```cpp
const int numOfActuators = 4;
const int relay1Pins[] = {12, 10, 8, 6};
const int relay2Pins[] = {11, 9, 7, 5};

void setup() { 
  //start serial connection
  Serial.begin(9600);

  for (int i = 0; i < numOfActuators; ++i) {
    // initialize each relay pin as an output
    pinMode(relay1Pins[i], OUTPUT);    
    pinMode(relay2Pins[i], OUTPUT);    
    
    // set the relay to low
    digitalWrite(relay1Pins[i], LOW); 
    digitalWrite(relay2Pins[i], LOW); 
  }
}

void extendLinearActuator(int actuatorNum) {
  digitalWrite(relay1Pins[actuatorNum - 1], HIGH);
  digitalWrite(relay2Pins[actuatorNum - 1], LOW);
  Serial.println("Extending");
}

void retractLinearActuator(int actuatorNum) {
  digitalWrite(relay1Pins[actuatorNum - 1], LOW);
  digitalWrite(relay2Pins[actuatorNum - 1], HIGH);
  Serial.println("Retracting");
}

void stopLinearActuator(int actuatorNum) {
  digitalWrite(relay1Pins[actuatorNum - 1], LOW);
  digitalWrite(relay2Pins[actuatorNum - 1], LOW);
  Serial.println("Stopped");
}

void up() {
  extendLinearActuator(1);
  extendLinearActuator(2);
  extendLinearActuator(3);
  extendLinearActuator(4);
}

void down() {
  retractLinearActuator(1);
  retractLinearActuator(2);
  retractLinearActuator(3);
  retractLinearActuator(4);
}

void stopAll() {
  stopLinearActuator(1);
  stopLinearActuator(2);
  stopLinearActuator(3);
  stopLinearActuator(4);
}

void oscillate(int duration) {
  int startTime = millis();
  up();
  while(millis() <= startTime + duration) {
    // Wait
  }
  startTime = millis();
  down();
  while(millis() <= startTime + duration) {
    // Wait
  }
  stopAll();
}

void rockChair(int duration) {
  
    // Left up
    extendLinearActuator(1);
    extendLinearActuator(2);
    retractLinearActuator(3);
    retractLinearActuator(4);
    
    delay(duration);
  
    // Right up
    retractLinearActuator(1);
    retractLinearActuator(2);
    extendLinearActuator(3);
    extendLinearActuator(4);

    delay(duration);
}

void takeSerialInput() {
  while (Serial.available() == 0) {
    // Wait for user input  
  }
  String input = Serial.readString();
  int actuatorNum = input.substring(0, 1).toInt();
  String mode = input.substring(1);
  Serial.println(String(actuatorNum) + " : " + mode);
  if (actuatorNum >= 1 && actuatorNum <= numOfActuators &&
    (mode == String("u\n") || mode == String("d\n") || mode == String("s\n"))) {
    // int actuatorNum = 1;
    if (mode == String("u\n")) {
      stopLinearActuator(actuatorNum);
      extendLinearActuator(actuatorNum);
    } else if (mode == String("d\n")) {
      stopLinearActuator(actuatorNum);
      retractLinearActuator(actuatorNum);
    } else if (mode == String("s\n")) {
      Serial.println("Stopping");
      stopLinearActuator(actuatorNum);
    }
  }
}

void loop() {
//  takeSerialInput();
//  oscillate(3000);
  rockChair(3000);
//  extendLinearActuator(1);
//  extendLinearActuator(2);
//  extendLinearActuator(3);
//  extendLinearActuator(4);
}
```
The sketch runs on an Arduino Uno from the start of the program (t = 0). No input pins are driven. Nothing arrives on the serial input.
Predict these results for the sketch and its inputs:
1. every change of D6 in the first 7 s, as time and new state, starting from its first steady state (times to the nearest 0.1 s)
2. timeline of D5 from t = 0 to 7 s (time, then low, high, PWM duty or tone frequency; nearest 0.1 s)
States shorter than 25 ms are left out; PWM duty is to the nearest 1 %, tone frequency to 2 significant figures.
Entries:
0 s low; 3 s high; 6 s low
0 s high; 3 s low; 6 s high
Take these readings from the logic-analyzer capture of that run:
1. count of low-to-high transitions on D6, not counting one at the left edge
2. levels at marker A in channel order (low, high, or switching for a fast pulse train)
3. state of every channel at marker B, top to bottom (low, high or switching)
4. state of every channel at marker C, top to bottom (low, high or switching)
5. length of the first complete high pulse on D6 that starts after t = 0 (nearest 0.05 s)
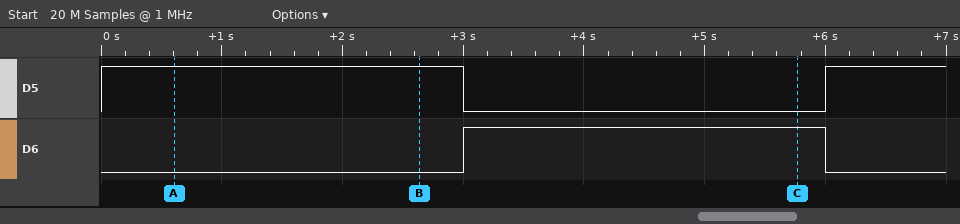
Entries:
1
D5 high, D6 low
D5 high, D6 low
D5 low, D6 high
3.00 s
